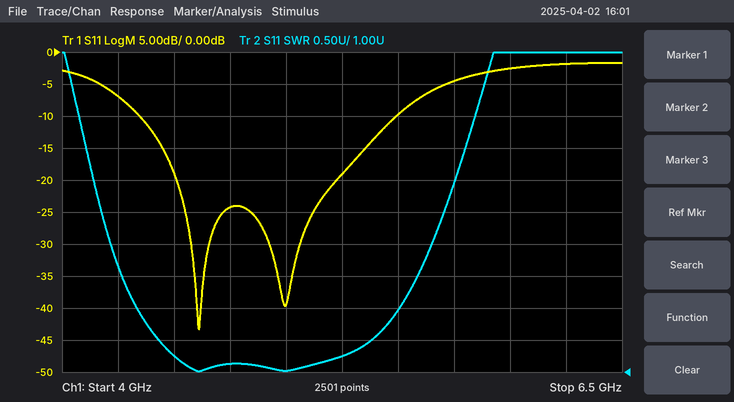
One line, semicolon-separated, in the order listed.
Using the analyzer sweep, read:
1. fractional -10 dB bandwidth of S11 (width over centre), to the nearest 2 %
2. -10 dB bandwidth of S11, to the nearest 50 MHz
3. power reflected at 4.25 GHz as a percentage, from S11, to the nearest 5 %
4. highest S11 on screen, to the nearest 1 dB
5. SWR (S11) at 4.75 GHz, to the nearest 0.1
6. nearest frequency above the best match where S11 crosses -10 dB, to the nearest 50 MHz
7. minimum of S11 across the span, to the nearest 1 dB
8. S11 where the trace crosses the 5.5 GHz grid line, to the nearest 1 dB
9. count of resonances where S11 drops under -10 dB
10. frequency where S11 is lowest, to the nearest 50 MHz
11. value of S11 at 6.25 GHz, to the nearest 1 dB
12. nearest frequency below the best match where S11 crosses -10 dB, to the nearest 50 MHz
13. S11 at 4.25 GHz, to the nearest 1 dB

24 %; 1.15 GHz; 20 %; -2 dB; 1.1; 5.50 GHz; -43 dB; -10 dB; 2; 4.60 GHz; -2 dB; 4.35 GHz; -7 dB
